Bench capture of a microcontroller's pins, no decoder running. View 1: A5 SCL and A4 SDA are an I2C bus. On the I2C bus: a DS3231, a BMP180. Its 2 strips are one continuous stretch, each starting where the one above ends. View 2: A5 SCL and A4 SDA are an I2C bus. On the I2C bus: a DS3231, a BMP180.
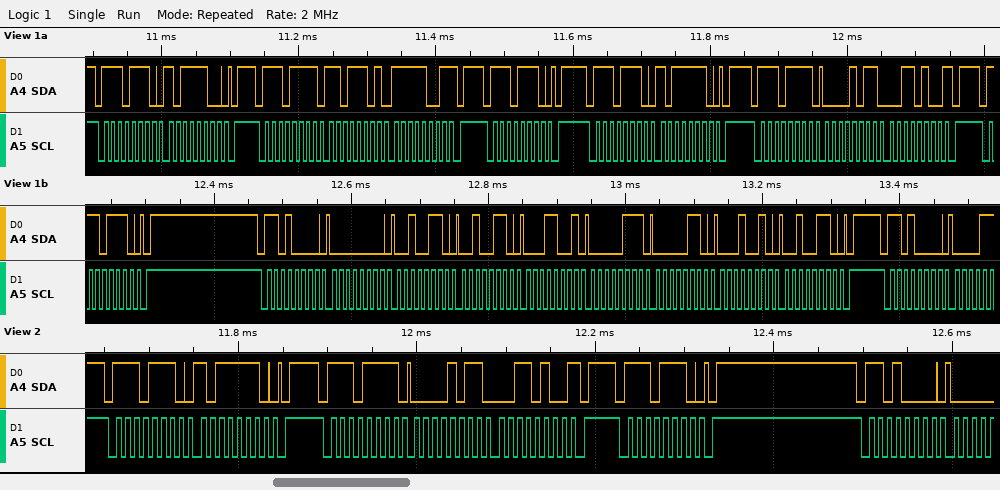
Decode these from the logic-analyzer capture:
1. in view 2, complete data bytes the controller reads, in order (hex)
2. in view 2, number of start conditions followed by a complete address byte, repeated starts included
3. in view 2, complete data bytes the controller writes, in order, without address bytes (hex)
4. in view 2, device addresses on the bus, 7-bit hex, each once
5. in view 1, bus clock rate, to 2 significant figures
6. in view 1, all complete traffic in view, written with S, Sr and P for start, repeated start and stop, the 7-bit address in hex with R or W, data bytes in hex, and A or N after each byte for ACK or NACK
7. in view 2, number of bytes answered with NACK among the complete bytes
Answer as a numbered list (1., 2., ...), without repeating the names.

1. 0B 34
2. 4
3. BE
4. 0x77 0x68
5. 100 kHz
6. S 77W A BC A P S 77R A DD A F9 N P S 77W A P S 77W A BE A P S 77R A 0B A 34 N P S 77W A P S 68W A 00 A 26 A 26 A 19 A 07 A 06 A 12 A 26 A P S 68W A
7. 1
